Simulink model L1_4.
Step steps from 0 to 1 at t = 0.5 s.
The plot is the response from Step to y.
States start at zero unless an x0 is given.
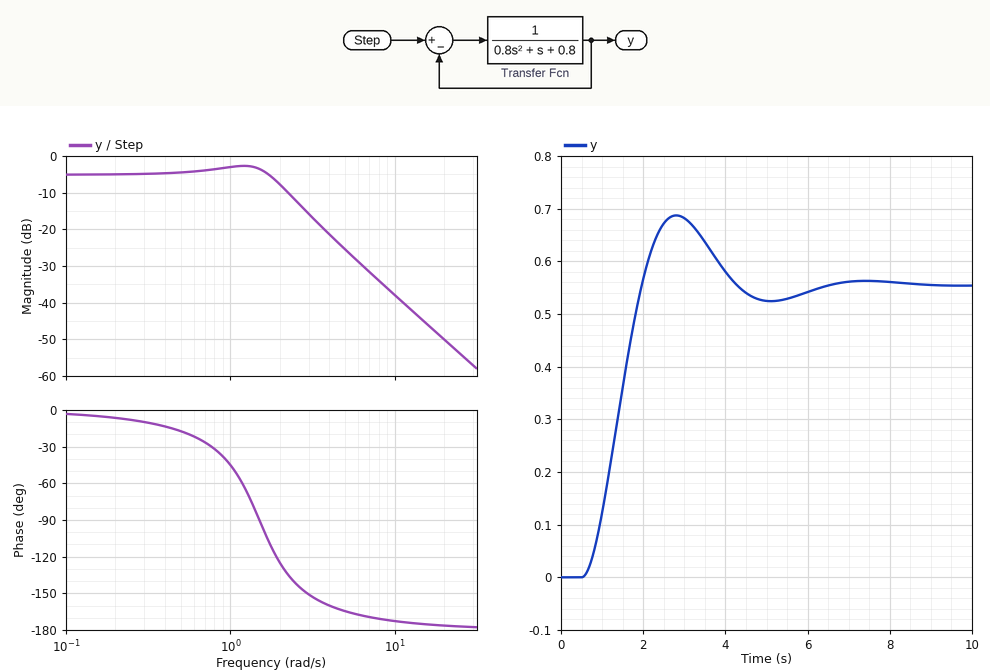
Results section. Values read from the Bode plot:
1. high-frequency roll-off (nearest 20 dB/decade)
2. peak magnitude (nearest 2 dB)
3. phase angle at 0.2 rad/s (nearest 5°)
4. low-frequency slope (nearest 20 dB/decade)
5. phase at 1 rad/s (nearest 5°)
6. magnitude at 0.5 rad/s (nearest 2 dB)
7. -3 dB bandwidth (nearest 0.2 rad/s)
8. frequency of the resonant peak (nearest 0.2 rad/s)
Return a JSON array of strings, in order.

["-40 dB/decade", "-2 dB", "-5°", "0 dB/decade", "-45°", "-4 dB", "2.0 rad/s", "1.2 rad/s"]
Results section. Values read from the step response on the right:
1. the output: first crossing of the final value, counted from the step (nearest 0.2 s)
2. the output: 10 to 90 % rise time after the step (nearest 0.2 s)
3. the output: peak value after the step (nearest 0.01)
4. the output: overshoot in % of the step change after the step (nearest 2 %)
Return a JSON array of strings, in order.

["1.4 s", "1.0 s", "0.69", "24 %"]
